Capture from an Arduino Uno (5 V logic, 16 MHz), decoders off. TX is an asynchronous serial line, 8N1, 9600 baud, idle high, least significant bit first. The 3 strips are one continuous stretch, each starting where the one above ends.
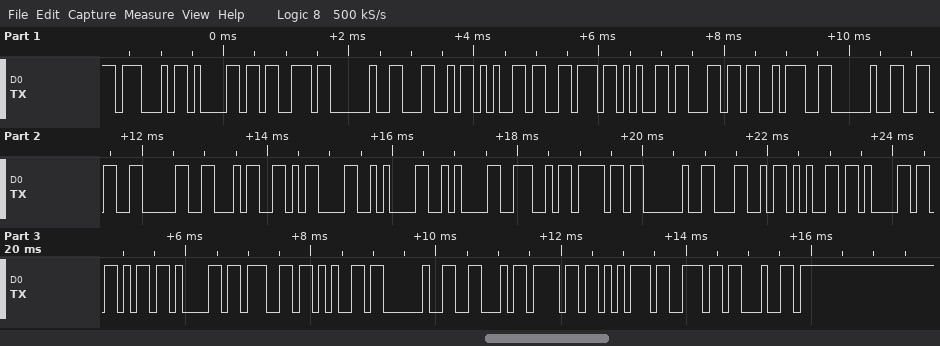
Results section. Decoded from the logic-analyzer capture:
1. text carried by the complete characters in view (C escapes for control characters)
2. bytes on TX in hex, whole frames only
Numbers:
"Gas Level: 604\r\n\nNo Leakage Found"
47 61 73 20 4C 65 76 65 6C 3A 20 36 30 34 0D 0A 0A 4E 6F 20 4C 65 61 6B 61 67 65 20 46 6F 75 6E 64
